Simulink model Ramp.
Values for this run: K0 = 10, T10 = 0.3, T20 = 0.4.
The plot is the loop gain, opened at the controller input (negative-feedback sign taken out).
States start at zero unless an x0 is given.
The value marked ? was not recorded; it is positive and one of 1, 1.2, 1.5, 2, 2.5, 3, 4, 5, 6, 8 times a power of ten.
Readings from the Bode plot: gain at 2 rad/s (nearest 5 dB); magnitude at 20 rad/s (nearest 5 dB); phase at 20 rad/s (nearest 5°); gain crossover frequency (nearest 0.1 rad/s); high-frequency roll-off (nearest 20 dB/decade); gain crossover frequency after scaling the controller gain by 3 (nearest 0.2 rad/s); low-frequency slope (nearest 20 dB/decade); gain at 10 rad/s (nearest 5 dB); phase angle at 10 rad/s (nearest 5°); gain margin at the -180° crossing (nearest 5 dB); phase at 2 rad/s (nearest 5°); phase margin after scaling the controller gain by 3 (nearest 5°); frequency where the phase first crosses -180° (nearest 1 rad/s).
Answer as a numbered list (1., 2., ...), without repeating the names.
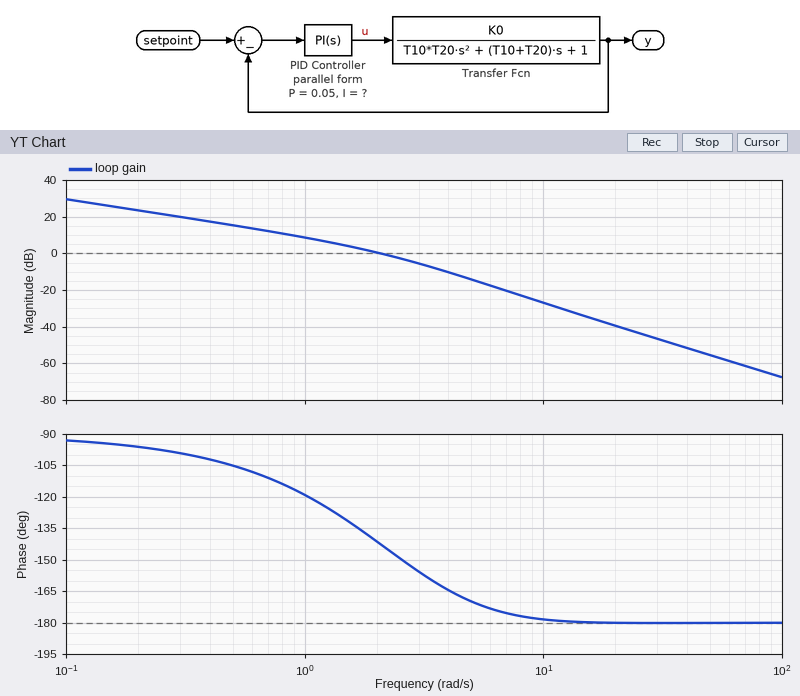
1. 0 dB
2. -40 dB
3. -180°
4. 2.1 rad/s
5. -40 dB/decade
6. 3.8 rad/s
7. -20 dB/decade
8. -25 dB
9. -180°
10. 35 dB
11. -140°
12. 15°
13. 17 rad/s
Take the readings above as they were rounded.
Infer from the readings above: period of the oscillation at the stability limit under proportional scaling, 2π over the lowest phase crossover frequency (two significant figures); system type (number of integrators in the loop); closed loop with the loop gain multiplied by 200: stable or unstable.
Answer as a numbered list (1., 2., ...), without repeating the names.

1. 0.37 s
2. 1
3. unstable
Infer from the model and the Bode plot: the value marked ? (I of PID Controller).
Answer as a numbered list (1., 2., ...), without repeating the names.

1. 0.3
